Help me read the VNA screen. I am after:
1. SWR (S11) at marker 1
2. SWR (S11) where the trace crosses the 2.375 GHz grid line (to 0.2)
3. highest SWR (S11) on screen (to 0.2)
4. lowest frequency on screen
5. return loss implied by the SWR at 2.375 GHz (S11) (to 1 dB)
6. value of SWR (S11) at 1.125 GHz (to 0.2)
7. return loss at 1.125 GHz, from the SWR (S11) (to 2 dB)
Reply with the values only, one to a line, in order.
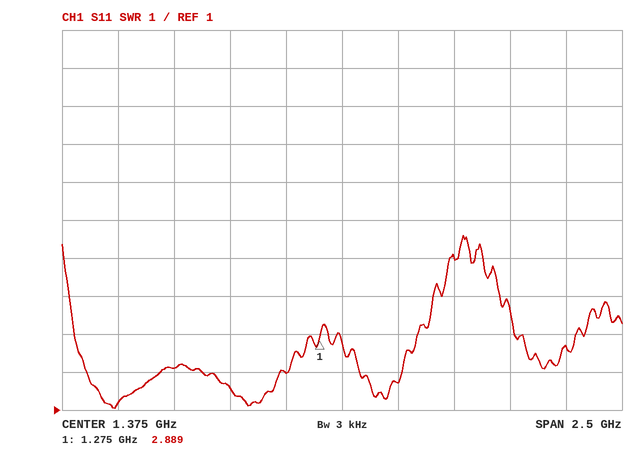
2.889
2.6
5.6
125 MHz
7 dB
2.0
10 dB
